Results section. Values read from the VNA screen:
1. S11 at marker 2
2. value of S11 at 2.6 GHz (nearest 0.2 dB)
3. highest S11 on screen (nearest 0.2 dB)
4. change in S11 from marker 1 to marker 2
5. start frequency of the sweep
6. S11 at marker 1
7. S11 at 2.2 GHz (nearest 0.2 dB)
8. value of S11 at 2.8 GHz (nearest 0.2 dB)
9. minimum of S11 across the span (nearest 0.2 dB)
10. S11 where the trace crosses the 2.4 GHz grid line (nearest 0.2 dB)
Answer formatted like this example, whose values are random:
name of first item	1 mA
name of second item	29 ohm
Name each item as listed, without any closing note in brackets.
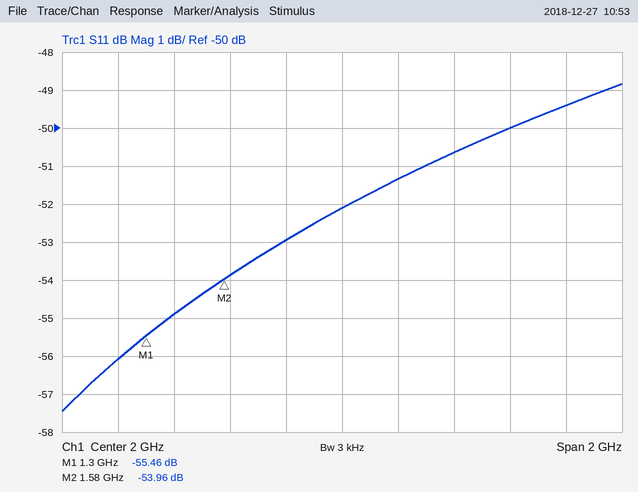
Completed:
S11 at marker 2	-53.96 dB
value of S11 at 2.6 GHz	-50.0 dB
highest S11 on screen	-48.8 dB
change in S11 from marker 1 to marker 2	1.50 dB
start frequency of the sweep	1 GHz
S11 at marker 1	-55.46 dB
S11 at 2.2 GHz	-51.4 dB
value of S11 at 2.8 GHz	-49.4 dB
minimum of S11 across the span	-57.4 dB
S11 where the trace crosses the 2.4 GHz grid line	-50.6 dB
